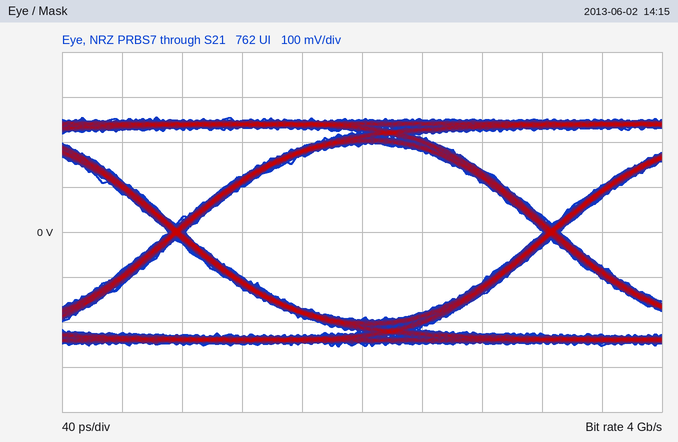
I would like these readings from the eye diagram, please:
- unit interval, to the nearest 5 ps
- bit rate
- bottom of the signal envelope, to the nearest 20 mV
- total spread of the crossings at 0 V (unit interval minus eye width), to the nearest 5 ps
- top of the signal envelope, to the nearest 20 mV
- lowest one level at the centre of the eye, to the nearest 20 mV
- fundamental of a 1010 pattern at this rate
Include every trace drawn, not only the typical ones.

250 ps
4 Gb/s
-260 mV
10 ps
260 mV
200 mV
2 GHz
